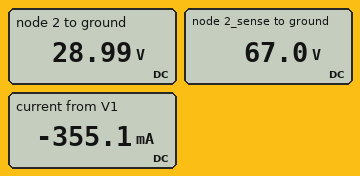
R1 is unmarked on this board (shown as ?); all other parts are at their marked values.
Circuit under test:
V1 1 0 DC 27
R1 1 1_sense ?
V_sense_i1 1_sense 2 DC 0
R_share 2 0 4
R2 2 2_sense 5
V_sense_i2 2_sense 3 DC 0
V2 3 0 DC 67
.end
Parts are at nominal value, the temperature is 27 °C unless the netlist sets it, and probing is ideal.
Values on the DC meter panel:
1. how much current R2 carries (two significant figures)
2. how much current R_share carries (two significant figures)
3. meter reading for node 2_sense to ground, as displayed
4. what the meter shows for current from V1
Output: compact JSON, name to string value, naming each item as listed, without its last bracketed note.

{"how much current R2 carries": "7.6 A", "how much current R_share carries": "7.2 A", "meter reading for node 2_sense to ground, as displayed": "67.0 V", "what the meter shows for current from V1": "-355.1 mA"}
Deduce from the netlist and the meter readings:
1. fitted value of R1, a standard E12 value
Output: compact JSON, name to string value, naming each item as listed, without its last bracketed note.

{"fitted value of R1, a standard E12 value": "5.6 Ω"}
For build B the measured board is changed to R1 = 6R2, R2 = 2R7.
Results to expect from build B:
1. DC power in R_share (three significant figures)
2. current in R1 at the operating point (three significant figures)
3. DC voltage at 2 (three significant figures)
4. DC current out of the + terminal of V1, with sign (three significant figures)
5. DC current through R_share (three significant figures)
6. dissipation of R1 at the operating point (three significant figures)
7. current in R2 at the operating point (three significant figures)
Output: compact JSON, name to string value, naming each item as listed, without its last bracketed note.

{"DC power in R_share": "348 W", "current in R1 at the operating point": "1.66 A", "DC voltage at 2": "37.3 V", "DC current out of the + terminal of V1, with sign": "-1.66 A", "DC current through R_share": "9.33 A", "dissipation of R1 at the operating point": "17.2 W", "current in R2 at the operating point": "11.0 A"}
